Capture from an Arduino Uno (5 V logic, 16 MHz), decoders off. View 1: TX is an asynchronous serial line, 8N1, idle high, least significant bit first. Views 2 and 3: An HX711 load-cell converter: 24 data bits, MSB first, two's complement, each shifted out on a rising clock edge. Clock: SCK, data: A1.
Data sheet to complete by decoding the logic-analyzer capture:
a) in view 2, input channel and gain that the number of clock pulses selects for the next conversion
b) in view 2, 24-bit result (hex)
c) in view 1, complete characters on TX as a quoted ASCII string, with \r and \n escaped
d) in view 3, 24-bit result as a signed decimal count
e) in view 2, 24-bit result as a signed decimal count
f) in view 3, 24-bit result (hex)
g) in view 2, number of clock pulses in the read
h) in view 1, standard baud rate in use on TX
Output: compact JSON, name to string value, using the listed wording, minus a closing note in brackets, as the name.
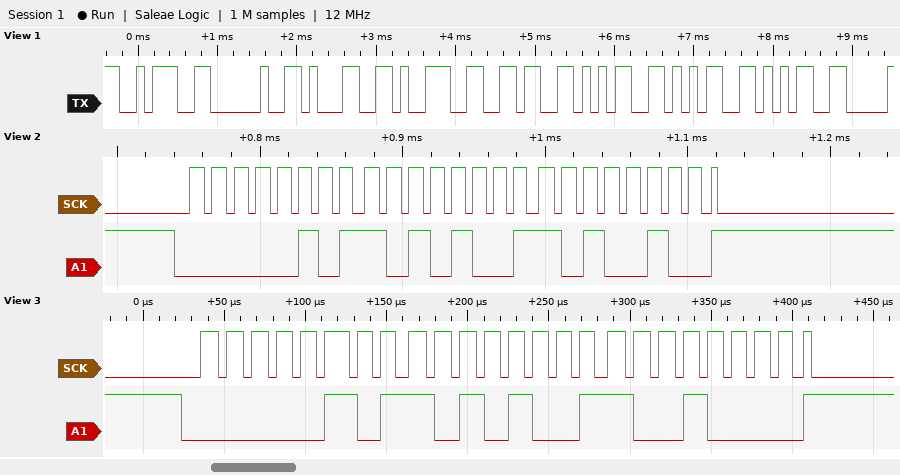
{"in view 2, input channel and gain that the number of clock pulses selects for the next conversion": "channel A, gain 128", "in view 2, 24-bit result": "0x05A9A4", "in view 1, complete characters on TX as a quoted ASCII string, with \\r and \\n escaped": "\": 196555\"", "in view 3, 24-bit result as a signed decimal count": "371088", "in view 2, 24-bit result as a signed decimal count": "371108", "in view 3, 24-bit result": "0x05A990", "in view 2, number of clock pulses in the read": "25", "in view 1, standard baud rate in use on TX": "9600 baud"}
